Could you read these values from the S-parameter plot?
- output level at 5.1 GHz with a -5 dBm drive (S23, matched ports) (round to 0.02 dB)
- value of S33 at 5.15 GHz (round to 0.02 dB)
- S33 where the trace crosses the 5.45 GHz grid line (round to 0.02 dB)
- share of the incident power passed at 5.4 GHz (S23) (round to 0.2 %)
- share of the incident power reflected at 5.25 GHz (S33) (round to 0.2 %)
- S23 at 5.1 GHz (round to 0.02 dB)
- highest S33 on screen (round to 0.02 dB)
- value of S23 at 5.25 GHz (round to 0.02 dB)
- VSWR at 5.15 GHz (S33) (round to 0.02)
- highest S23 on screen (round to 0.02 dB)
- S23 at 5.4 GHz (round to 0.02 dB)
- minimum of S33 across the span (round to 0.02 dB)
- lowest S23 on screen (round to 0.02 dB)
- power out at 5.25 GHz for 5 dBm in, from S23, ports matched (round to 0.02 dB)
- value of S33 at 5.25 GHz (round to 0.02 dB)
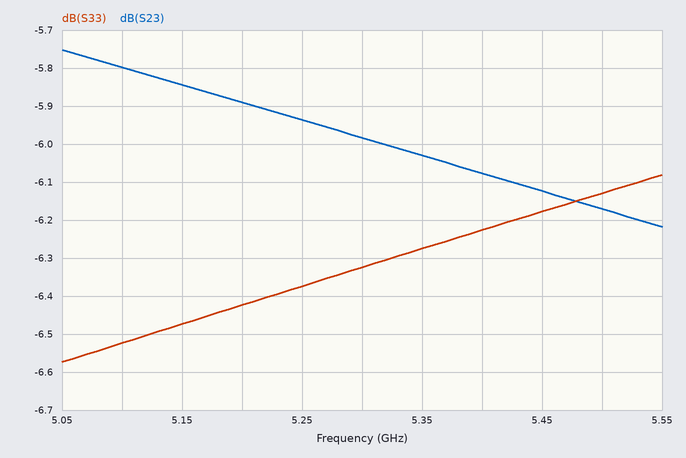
-10.80 dBm
-6.48 dB
-6.18 dB
24.6 %
23.0 %
-5.80 dB
-6.08 dB
-5.94 dB
2.80
-5.76 dB
-6.08 dB
-6.58 dB
-6.22 dB
-0.94 dBm
-6.38 dB
